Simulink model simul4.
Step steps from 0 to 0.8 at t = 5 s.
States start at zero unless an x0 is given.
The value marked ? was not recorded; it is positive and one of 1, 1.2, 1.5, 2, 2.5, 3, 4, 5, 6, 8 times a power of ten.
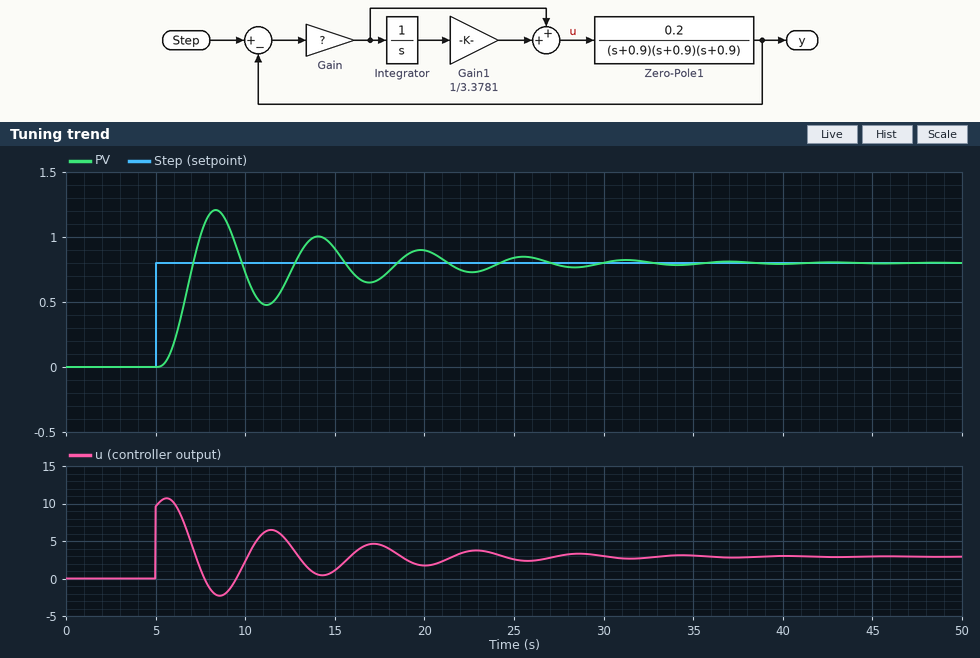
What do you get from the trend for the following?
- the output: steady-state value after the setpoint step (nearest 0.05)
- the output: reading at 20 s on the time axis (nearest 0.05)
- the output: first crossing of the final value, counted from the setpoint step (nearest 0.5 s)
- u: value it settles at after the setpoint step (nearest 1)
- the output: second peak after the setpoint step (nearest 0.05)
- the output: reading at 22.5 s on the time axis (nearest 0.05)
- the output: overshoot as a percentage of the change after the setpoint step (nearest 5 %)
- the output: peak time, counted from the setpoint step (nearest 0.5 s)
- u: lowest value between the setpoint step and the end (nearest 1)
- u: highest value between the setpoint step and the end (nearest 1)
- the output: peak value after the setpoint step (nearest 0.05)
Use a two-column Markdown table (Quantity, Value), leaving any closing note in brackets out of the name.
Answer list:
| Quantity | Value |
|---|---|
| the output: steady-state value after the setpoint step | 0.80 |
| the output: reading at 20 s on the time axis | 0.90 |
| the output: first crossing of the final value, counted from the setpoint step | 2.0 s |
| u: value it settles at after the setpoint step | 3 |
| the output: second peak after the setpoint step | 1.00 |
| the output: reading at 22.5 s on the time axis | 0.75 |
| the output: overshoot as a percentage of the change after the setpoint step | 50 % |
| the output: peak time, counted from the setpoint step | 3.5 s |
| u: lowest value between the setpoint step and the end | -2 |
| u: highest value between the setpoint step and the end | 11 |
| the output: peak value after the setpoint step | 1.20 |
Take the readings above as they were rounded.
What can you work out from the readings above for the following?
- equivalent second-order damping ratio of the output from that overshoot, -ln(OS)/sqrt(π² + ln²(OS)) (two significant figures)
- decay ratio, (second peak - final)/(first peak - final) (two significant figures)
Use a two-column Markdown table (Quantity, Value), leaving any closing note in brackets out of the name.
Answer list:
| Quantity | Value |
|---|---|
| equivalent second-order damping ratio of the output from that overshoot, -ln(OS)/sqrt(π² + ln²(OS)) | 0.22 |
| decay ratio, (second peak - final)/(first peak - final) | 0.50 |
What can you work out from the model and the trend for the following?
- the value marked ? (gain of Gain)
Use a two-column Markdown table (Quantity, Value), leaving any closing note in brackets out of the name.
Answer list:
| Quantity | Value |
|---|---|
| the value marked ? | 12 |
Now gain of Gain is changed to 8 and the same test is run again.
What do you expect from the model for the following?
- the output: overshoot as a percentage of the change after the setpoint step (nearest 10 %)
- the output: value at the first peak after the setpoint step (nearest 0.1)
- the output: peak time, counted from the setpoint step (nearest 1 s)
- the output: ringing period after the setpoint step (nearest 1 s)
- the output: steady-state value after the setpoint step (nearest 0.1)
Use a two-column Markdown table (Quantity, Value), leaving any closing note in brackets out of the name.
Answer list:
| Quantity | Value |
|---|---|
| the output: overshoot as a percentage of the change after the setpoint step | 30 % |
| the output: value at the first peak after the setpoint step | 1.0 |
| the output: peak time, counted from the setpoint step | 4 s |
| the output: ringing period after the setpoint step | 7 s |
| the output: steady-state value after the setpoint step | 0.8 |
